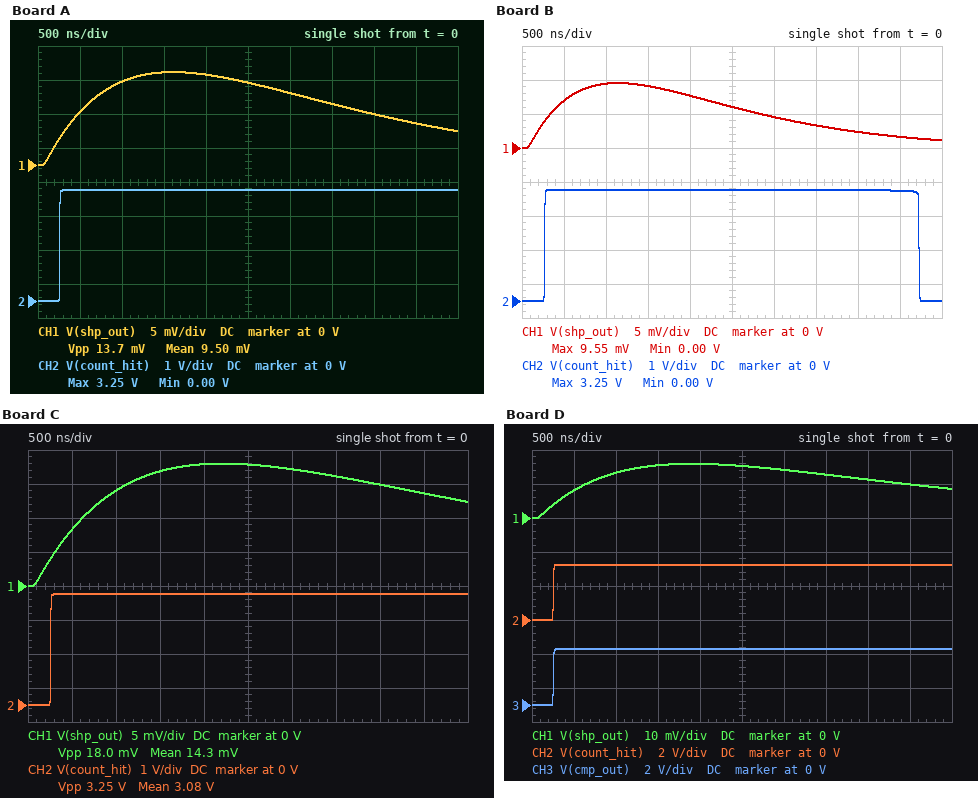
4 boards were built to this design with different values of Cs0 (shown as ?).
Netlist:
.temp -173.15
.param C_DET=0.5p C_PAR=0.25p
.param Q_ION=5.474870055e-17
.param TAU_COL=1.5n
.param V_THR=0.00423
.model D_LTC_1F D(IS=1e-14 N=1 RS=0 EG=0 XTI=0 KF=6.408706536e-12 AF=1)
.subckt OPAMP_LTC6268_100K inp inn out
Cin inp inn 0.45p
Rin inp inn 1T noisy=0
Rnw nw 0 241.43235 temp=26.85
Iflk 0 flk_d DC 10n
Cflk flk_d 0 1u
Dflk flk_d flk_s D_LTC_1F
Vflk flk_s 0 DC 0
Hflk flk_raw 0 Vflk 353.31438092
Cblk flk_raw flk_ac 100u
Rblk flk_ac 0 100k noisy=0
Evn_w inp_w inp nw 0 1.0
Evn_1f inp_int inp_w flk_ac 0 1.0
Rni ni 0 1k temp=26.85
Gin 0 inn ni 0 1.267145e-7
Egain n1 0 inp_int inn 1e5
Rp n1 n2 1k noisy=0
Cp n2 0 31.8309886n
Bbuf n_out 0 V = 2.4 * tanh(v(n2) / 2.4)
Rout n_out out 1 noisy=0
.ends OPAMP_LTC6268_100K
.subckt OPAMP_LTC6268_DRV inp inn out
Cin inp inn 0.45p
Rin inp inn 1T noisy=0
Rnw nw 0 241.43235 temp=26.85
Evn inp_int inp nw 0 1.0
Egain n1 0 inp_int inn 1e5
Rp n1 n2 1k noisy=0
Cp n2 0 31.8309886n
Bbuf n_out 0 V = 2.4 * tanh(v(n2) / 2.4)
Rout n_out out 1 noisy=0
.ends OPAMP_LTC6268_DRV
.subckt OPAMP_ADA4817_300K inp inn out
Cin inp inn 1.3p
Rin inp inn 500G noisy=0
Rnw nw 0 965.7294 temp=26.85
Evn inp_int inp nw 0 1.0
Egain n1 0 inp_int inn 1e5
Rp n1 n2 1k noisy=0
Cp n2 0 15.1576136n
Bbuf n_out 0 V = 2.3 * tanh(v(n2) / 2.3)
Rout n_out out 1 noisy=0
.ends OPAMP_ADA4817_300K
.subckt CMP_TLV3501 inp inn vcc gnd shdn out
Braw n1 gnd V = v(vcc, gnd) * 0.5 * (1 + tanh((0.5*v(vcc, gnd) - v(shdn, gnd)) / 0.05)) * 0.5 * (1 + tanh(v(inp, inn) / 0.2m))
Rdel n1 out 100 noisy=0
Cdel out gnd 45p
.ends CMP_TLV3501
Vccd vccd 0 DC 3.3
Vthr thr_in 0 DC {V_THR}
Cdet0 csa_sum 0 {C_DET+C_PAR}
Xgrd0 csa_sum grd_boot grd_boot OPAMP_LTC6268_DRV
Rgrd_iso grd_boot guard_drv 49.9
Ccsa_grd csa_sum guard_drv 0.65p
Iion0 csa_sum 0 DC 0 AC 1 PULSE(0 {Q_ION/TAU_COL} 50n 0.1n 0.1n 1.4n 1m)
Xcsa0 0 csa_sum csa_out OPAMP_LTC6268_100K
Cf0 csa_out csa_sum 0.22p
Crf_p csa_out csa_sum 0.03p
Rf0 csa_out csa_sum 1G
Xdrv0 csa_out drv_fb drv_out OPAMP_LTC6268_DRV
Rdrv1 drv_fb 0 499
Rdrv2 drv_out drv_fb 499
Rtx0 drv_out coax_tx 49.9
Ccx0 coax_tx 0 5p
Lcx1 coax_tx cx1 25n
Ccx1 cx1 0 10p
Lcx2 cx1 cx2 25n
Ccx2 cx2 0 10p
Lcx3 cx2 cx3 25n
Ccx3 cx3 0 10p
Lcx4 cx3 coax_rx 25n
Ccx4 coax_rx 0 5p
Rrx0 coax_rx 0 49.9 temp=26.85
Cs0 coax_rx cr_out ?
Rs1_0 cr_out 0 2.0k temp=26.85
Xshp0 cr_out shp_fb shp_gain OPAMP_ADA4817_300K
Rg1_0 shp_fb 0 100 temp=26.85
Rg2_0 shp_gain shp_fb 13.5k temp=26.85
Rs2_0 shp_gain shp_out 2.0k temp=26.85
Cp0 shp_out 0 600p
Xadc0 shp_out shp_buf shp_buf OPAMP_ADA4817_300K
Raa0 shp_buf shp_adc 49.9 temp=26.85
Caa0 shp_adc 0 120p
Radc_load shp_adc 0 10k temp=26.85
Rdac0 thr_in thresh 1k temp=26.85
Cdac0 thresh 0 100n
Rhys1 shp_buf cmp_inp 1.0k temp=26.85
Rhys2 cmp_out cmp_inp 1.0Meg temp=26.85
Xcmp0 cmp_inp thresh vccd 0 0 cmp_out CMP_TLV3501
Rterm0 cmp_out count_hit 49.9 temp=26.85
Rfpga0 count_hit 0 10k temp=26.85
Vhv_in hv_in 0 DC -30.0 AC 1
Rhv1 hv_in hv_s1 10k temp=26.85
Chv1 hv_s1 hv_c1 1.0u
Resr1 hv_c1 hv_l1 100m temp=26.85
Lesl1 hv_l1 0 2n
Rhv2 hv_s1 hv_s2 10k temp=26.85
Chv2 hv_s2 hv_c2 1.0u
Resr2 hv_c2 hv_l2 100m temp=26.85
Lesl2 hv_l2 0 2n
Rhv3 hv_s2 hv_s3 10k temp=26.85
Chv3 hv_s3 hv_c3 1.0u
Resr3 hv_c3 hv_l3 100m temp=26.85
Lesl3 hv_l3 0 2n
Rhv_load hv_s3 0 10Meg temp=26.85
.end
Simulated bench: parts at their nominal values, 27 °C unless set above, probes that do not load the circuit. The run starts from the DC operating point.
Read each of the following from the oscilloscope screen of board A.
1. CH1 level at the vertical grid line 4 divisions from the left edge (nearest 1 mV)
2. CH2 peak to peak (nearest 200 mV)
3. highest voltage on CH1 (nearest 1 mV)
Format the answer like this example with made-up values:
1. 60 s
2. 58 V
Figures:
1. 13 mV
2. 3.2 V
3. 14 mV
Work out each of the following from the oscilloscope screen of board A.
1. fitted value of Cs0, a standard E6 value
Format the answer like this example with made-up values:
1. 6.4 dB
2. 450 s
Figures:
1. 1 nF
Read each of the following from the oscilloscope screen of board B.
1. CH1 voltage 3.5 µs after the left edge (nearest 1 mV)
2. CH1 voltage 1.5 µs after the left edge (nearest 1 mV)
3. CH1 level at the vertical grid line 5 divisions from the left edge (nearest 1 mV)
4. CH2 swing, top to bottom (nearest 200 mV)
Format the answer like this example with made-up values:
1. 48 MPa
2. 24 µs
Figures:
1. 3 mV
2. 9 mV
3. 6 mV
4. 3.2 V
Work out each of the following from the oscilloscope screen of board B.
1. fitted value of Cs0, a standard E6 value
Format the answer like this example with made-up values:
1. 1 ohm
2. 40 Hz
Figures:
1. 470 pF
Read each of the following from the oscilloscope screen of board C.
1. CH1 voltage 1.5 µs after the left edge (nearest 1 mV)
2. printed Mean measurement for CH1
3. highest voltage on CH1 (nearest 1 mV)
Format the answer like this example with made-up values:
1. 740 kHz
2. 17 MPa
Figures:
1. 17 mV
2. 14.3 mV
3. 18 mV
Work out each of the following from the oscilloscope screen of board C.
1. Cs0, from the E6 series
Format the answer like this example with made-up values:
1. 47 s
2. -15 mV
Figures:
1. 2.2 nF
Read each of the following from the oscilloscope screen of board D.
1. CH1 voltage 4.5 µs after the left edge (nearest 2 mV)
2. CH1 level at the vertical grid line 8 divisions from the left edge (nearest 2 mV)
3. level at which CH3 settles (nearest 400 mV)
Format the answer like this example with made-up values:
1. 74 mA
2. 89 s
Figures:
1. 10 mV
2. 12 mV
3. 3.2 V
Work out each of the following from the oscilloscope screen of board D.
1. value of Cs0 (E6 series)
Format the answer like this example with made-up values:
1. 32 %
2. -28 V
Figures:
1. 1.5 nF
